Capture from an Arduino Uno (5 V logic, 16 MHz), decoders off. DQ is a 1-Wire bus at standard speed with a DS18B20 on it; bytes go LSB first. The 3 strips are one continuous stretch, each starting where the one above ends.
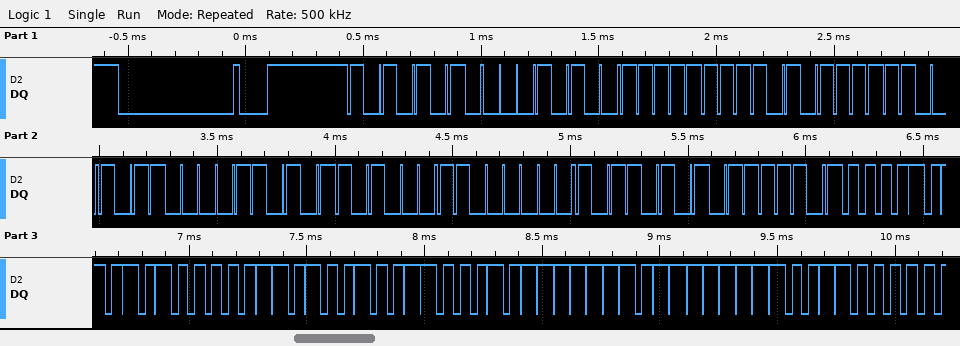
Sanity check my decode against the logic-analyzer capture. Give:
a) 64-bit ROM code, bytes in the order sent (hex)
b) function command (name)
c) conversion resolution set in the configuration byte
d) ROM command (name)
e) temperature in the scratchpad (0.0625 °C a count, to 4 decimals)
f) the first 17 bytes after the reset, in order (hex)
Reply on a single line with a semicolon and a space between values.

28 FF F5 D3 B0 16 03 AD; Read Scratchpad; 12 bits; Match ROM; 85.0000 °C; 55 28 FF F5 D3 B0 16 03 AD BE 50 05 4B 46 7F FF 0C
